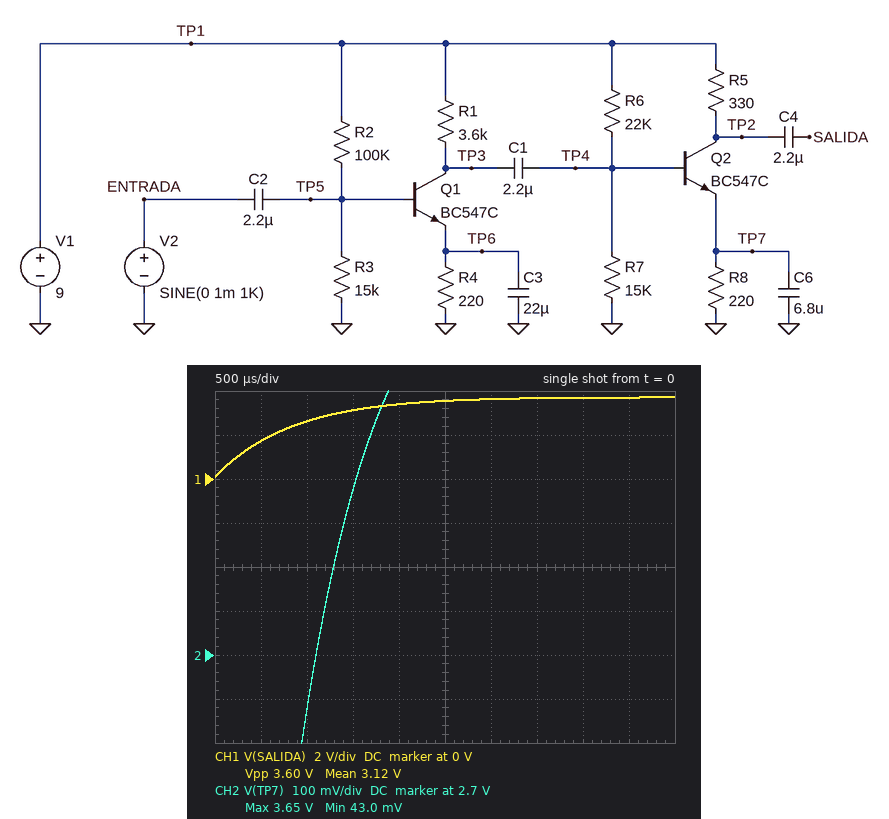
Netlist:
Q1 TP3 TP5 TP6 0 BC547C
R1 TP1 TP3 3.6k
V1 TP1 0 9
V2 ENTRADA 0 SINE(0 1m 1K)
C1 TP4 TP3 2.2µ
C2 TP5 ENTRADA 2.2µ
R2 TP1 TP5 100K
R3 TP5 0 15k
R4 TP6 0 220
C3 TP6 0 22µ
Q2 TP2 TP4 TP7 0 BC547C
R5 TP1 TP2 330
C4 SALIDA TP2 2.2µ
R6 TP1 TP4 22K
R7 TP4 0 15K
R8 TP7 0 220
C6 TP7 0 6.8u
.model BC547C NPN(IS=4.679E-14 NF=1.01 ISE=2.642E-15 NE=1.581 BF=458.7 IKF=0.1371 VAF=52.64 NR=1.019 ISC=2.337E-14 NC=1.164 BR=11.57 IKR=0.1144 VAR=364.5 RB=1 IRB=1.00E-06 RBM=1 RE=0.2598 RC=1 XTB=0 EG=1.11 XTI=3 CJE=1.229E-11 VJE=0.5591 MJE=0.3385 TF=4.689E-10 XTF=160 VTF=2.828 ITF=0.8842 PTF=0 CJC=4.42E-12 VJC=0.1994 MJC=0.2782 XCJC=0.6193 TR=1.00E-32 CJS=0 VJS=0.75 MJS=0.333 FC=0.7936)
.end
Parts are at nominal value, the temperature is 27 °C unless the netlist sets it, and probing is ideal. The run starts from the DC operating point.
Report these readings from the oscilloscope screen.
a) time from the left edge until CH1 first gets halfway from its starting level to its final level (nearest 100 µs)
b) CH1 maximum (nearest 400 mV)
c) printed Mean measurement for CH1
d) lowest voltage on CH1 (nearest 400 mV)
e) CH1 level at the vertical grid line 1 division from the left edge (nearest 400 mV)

600 µs
3.6 V
3.12 V
0 V
1.6 V
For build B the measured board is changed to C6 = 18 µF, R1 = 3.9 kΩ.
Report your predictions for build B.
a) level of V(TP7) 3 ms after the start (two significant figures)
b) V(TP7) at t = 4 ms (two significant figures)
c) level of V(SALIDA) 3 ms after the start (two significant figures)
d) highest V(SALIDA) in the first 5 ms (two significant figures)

2.7 V
3.0 V
2.8 V
3.3 V
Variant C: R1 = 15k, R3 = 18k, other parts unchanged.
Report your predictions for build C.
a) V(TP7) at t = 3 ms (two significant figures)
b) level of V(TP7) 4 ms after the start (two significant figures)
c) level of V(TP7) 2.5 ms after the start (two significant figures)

3.5 V
3.6 V
3.4 V
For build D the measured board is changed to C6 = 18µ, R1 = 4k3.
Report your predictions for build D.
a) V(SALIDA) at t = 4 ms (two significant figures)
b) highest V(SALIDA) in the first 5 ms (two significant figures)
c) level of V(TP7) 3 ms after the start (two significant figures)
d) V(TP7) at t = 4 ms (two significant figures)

3.1 V
3.3 V
2.7 V
3.0 V
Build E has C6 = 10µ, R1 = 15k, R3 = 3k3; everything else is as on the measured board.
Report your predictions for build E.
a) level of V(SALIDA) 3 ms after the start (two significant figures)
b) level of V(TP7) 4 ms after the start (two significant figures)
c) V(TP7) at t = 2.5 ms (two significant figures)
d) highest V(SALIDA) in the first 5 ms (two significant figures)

3.3 V
3.4 V
3.1 V
3.6 V
